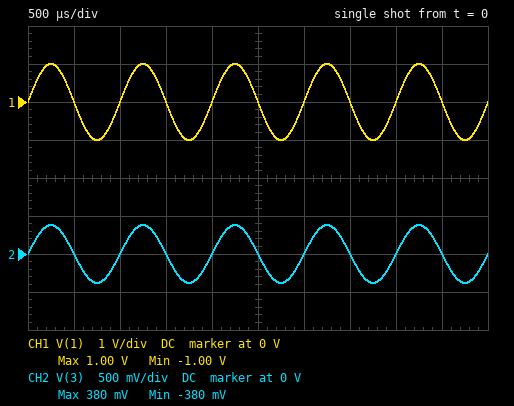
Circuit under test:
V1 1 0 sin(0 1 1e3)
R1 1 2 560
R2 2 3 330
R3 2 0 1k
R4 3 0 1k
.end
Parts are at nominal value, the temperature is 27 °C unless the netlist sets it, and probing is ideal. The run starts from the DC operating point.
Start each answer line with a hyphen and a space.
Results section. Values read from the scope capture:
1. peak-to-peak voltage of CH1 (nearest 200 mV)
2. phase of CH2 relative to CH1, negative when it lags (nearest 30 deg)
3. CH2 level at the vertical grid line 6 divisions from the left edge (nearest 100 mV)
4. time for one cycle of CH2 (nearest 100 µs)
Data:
- 2.0 V
- 0 deg
- 0 V
- 1.0 ms
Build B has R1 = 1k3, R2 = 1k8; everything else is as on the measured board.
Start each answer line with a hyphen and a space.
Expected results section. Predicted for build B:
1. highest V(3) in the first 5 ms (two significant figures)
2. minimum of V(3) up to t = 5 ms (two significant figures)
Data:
- 130 mV
- -130 mV
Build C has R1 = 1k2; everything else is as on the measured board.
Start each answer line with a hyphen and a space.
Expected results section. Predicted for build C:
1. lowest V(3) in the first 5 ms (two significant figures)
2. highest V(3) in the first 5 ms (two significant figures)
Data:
- -240 mV
- 240 mV
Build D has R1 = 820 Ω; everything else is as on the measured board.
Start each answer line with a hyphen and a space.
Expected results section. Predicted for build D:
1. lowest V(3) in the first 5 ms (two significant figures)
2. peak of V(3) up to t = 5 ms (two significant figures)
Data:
- -310 mV
- 310 mV
